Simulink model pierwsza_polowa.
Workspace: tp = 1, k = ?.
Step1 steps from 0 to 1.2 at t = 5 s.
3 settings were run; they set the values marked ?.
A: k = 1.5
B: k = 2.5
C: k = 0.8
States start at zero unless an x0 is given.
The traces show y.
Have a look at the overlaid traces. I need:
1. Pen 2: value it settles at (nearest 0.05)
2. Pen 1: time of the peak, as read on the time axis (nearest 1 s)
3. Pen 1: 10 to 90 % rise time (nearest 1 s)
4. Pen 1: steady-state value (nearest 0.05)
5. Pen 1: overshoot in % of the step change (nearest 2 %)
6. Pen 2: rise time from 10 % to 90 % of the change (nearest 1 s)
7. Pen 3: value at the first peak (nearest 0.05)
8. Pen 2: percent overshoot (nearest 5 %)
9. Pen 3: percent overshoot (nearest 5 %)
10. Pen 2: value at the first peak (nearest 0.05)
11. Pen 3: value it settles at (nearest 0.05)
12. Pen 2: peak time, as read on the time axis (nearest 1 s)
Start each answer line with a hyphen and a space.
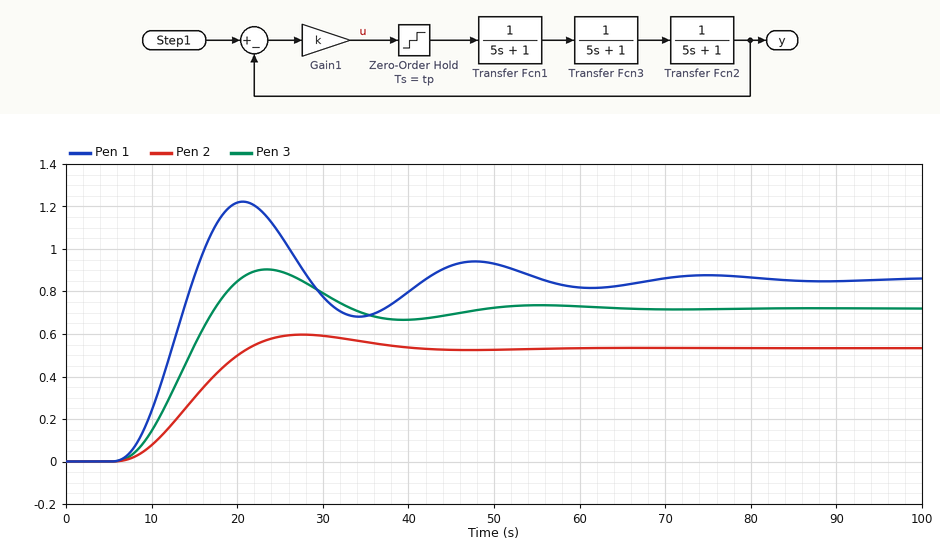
- 0.55
- 21 s
- 6 s
- 0.85
- 42 %
- 10 s
- 0.90
- 10 %
- 25 %
- 0.60
- 0.70
- 28 s
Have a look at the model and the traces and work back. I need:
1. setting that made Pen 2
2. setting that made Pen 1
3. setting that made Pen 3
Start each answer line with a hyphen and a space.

- C
- B
- A
